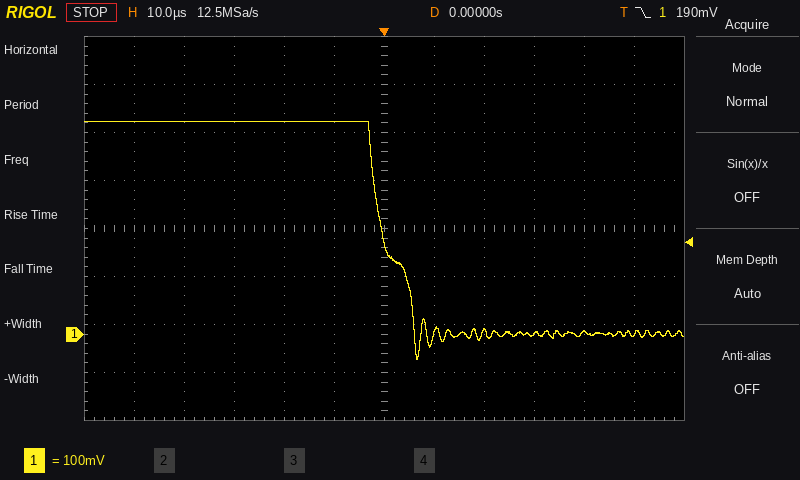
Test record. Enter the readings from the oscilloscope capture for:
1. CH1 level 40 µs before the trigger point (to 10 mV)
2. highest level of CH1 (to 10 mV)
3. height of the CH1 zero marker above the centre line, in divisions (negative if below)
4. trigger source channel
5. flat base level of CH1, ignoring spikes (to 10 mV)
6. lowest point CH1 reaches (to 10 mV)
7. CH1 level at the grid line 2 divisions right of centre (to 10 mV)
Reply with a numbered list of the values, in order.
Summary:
1. 440 mV
2. 440 mV
3. -2.2 div
4. CH1
5. 0 mV
6. -50 mV
7. 0 mV
